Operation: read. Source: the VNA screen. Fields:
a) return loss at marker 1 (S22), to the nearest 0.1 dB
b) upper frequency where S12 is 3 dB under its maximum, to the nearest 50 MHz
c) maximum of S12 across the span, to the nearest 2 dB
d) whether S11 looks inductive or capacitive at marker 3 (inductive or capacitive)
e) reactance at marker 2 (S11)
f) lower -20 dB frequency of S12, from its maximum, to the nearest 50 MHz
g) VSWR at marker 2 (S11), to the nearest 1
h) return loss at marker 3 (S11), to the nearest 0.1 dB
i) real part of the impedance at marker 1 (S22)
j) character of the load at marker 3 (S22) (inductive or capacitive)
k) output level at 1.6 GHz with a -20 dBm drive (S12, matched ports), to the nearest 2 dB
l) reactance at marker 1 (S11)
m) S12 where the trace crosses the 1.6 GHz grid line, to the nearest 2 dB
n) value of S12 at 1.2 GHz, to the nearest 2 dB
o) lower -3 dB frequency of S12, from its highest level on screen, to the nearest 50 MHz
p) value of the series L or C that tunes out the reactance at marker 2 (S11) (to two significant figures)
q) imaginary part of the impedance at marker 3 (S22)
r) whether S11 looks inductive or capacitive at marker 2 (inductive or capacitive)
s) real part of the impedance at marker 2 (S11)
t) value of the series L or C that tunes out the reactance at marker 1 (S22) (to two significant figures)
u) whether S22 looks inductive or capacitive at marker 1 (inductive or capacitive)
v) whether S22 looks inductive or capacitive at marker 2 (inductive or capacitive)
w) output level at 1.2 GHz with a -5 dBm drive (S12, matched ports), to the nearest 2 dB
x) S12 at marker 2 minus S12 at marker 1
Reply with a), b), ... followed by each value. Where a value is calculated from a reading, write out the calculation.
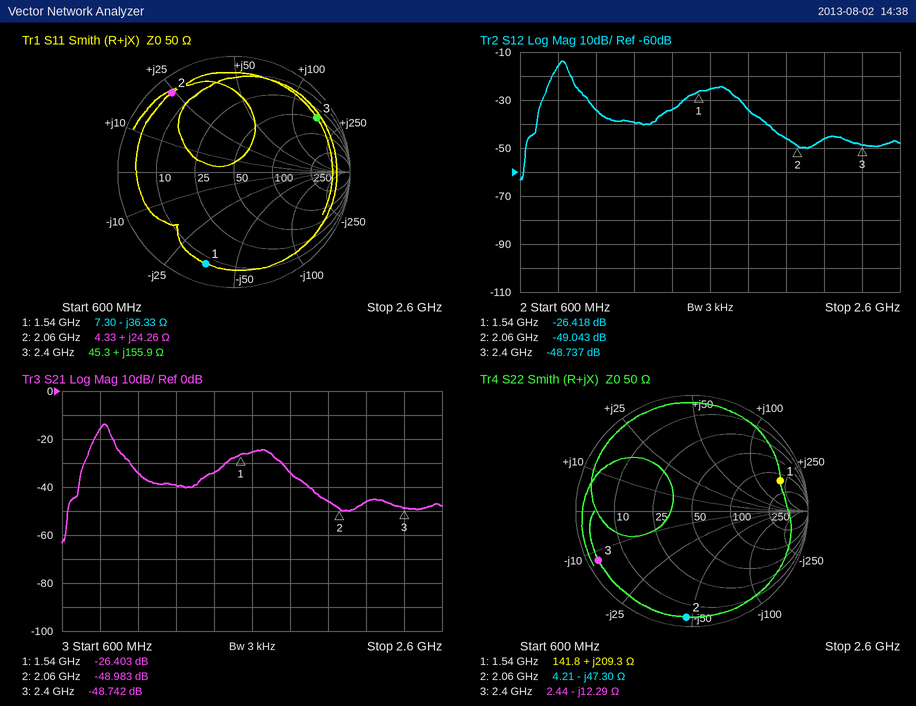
a) 1.9 dB
b) 850 MHz
c) -14 dB
d) inductive
e) +24.26 Ω
f) 700 MHz
g) 14
h) 1.4 dB
i) 141.8 Ω
j) capacitive
k) -20 dBm + (-26 dB) = -46 dBm
l) -36.33 Ω
m) -26 dB
n) -40 dB
o) 800 MHz
p) C = 1/(2π × 2.06 GHz × 24.26 Ω) ≈ 3.2 pF
q) -12.29 Ω
r) inductive
s) 4.33 Ω
t) C = 1/(2π × 1.54 GHz × 209.3 Ω) ≈ 494 fF, so 490 fF to two significant figures
u) inductive
v) capacitive
w) -5 dBm + (-40 dB) = -44 dBm
x) -49.043 − (-26.418) = -22.625 dB
